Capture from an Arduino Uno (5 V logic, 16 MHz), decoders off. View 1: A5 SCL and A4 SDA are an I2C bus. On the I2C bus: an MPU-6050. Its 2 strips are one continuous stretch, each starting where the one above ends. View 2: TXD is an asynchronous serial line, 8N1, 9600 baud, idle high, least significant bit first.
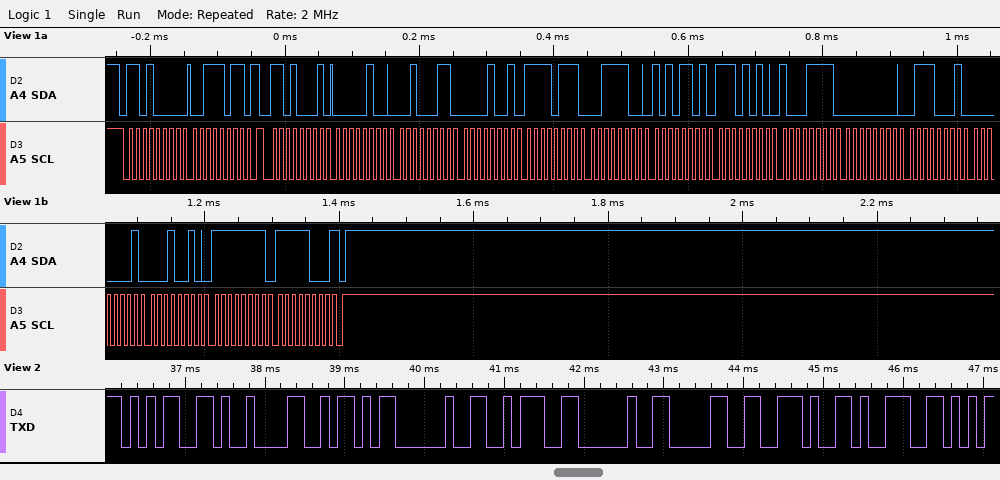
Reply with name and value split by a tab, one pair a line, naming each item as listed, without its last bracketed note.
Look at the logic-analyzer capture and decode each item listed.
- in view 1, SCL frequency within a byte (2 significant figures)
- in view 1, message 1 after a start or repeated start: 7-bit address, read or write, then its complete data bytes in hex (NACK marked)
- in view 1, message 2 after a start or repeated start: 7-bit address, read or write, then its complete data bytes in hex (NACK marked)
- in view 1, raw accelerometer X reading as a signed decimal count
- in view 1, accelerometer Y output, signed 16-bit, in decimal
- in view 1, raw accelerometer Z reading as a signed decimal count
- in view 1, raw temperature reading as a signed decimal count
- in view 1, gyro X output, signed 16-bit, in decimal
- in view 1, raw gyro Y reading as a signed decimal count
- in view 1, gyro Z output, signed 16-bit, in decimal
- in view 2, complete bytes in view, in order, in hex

in view 1, SCL frequency within a byte	100 kHz
in view 1, message 1 after a start or repeated start: 7-bit address, read or write, then its complete data bytes in hex	0x68 write: 3B
in view 1, message 2 after a start or repeated start: 7-bit address, read or write, then its complete data bytes in hex	0x68 read: 04 23 09 F7 3C AD EA 8F 00 71 01 12 FF F8 NACK
in view 1, raw accelerometer X reading as a signed decimal count	1059
in view 1, accelerometer Y output, signed 16-bit, in decimal	2551
in view 1, raw accelerometer Z reading as a signed decimal count	15533
in view 1, raw temperature reading as a signed decimal count	-5489
in view 1, gyro X output, signed 16-bit, in decimal	113
in view 1, raw gyro Y reading as a signed decimal count	274
in view 1, gyro Z output, signed 16-bit, in decimal	-8
in view 2, complete bytes in view, in order, in hex	0x35 0x09 0x5A 0x20 0x3A 0x20 0x30 0x2E 0x39
